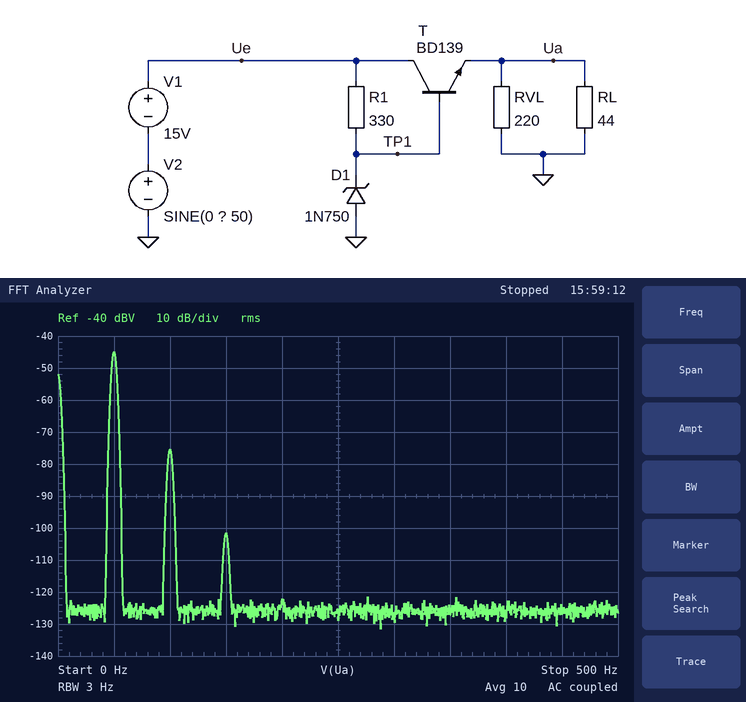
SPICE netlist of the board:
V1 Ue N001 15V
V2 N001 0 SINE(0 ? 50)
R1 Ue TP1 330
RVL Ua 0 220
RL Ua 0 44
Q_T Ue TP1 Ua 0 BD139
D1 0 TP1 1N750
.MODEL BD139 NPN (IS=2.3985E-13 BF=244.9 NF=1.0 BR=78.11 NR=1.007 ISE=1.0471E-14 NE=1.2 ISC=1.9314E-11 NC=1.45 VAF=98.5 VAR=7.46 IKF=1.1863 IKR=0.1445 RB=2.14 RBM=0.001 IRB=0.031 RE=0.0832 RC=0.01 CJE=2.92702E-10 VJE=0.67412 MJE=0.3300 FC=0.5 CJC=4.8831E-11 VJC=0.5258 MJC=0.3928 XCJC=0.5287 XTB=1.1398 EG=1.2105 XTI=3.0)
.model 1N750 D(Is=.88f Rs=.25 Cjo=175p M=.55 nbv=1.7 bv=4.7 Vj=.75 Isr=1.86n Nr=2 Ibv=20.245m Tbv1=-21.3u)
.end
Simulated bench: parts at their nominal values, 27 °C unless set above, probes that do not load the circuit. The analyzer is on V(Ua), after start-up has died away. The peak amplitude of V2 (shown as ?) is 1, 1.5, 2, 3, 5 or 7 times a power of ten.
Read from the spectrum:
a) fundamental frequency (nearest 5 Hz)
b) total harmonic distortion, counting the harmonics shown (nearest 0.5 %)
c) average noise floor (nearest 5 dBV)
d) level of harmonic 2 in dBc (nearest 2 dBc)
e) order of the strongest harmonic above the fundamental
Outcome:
50 Hz
3.0 %
-125 dBV
-30 dBc
2
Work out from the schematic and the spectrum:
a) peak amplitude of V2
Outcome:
1.5 V
